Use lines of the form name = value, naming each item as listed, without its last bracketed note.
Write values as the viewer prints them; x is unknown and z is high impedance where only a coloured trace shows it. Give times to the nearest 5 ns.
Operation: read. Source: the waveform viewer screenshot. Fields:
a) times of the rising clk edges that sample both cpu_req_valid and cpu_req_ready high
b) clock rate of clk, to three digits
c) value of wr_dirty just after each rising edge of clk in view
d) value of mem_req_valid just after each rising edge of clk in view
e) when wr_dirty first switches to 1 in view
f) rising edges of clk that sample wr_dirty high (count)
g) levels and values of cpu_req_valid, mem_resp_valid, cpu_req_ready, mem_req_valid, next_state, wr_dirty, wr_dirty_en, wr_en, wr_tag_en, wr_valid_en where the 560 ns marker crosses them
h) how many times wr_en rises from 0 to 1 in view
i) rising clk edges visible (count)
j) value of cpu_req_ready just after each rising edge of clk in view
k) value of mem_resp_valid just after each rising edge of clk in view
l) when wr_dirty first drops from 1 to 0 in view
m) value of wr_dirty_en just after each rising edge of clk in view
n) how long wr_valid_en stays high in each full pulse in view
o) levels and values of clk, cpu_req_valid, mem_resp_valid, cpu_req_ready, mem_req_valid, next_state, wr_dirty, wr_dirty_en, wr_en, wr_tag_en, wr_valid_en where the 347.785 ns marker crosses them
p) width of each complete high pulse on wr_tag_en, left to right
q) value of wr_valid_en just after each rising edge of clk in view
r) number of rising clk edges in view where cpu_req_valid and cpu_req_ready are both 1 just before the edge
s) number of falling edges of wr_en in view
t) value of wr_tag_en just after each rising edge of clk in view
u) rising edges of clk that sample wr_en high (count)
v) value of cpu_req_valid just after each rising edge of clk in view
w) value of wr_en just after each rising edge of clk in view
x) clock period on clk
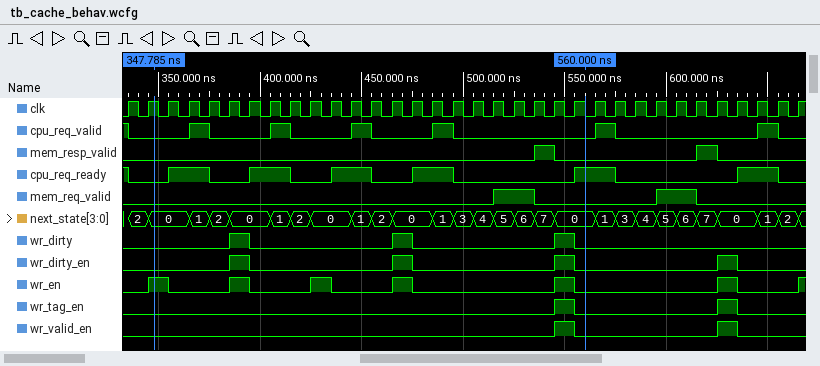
times of the rising clk edges that sample both cpu_req_valid and cpu_req_ready high = 335 ns, 375 ns, 415 ns, 455 ns, 495 ns, 575 ns, 655 ns
clock rate of clk, to three digits = 100 MHz
value of wr_dirty just after each rising edge of clk in view = 0 0 0 0 0 1 0 0 0 0 0 0 0 1 0 0 0 0 0 0 0 1 0 0 0 0 0 0 0 0 0 0 0 0
value of mem_req_valid just after each rising edge of clk in view = 0 0 0 0 0 0 0 0 0 0 0 0 0 0 0 0 0 0 1 1 0 0 0 0 0 0 1 1 0 0 0 0 0 0
when wr_dirty first switches to 1 in view = 385 ns
rising edges of clk that sample wr_dirty high = 3
levels and values of cpu_req_valid, mem_resp_valid, cpu_req_ready, mem_req_valid, next_state, wr_dirty, wr_dirty_en, wr_en, wr_tag_en, wr_valid_en where the 560 ns marker crosses them = cpu_req_valid=0, mem_resp_valid=0, cpu_req_ready=1, mem_req_valid=0, next_state=0, wr_dirty=0, wr_dirty_en=0, wr_en=0, wr_tag_en=0, wr_valid_en=0
how many times wr_en rises from 0 to 1 in view = 7
rising clk edges visible = 34
value of cpu_req_ready just after each rising edge of clk in view = 0 0 1 1 0 0 1 1 0 0 1 1 0 0 1 1 0 0 0 0 0 0 1 1 0 0 0 0 0 0 1 1 0 0
value of mem_resp_valid just after each rising edge of clk in view = 0 0 0 0 0 0 0 0 0 0 0 0 0 0 0 0 0 0 0 0 1 0 0 0 0 0 0 0 1 0 0 0 0 0
when wr_dirty first drops from 1 to 0 in view = 395 ns
value of wr_dirty_en just after each rising edge of clk in view = 0 0 0 0 0 1 0 0 0 0 0 0 0 1 0 0 0 0 0 0 0 1 0 0 0 0 0 0 0 1 0 0 0 0
how long wr_valid_en stays high in each full pulse in view = 10 ns, 10 ns
levels and values of clk, cpu_req_valid, mem_resp_valid, cpu_req_ready, mem_req_valid, next_state, wr_dirty, wr_dirty_en, wr_en, wr_tag_en, wr_valid_en where the 347.785 ns marker crosses them = clk=1, cpu_req_valid=0, mem_resp_valid=0, cpu_req_ready=0, mem_req_valid=0, next_state=0, wr_dirty=0, wr_dirty_en=0, wr_en=1, wr_tag_en=0, wr_valid_en=0
width of each complete high pulse on wr_tag_en, left to right = 10 ns, 10 ns
value of wr_valid_en just after each rising edge of clk in view = 0 0 0 0 0 0 0 0 0 0 0 0 0 0 0 0 0 0 0 0 0 1 0 0 0 0 0 0 0 1 0 0 0 0
number of rising clk edges in view where cpu_req_valid and cpu_req_ready are both 1 just before the edge = 7
number of falling edges of wr_en in view = 6
value of wr_tag_en just after each rising edge of clk in view = 0 0 0 0 0 0 0 0 0 0 0 0 0 0 0 0 0 0 0 0 0 1 0 0 0 0 0 0 0 1 0 0 0 0
rising edges of clk that sample wr_en high = 6
value of cpu_req_valid just after each rising edge of clk in view = 0 0 0 1 0 0 0 1 0 0 0 1 0 0 0 1 0 0 0 0 0 0 0 1 0 0 0 0 0 0 0 1 0 0
value of wr_en just after each rising edge of clk in view = 0 1 0 0 0 1 0 0 0 1 0 0 0 1 0 0 0 0 0 0 0 1 0 0 0 0 0 0 0 1 0 0 0 1
clock period on clk = 10 ns
